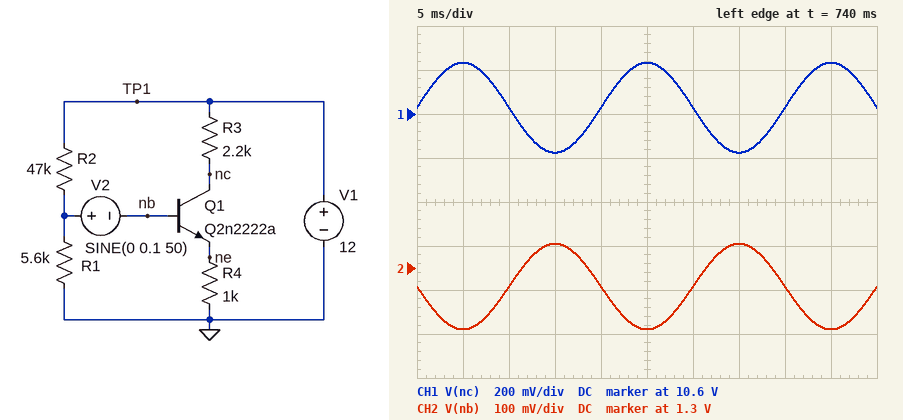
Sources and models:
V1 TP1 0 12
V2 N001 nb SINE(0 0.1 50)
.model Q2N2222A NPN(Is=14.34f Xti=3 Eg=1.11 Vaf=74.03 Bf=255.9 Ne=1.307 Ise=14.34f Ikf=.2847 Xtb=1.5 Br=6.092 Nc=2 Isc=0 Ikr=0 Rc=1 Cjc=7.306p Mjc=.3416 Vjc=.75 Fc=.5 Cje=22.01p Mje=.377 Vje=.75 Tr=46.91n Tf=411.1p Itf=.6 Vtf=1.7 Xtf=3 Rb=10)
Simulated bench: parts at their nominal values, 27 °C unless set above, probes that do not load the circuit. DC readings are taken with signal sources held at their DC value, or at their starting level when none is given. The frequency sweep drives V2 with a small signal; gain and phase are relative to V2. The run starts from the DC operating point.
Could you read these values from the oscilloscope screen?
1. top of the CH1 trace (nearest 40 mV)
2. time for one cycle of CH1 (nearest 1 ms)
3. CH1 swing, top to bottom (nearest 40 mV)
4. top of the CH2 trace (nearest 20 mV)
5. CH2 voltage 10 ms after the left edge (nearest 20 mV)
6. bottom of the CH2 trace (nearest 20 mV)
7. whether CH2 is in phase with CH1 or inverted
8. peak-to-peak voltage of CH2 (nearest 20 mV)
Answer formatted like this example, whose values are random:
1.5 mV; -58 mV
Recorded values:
10.84 V; 20 ms; 400 mV; 1.36 V; 1.26 V; 1.16 V; inverted; 200 mV
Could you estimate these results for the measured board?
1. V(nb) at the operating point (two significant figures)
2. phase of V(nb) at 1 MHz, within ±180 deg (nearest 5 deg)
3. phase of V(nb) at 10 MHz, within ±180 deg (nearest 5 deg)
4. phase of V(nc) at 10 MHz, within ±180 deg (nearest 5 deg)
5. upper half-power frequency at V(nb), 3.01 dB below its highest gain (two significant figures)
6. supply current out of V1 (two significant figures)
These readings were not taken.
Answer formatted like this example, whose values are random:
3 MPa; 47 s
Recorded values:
1.3 V; 160 deg; 130 deg; -90 deg; 2.6 MHz; 850 µA
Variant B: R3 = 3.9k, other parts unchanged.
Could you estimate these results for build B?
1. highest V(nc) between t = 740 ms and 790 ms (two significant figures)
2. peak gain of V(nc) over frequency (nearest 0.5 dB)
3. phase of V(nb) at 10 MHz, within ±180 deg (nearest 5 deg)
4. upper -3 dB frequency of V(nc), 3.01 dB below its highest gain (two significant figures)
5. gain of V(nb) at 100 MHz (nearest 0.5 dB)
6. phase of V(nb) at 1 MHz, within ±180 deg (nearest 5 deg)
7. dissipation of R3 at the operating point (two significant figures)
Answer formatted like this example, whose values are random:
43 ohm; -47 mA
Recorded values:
9.9 V; 11.0 dB; 140 deg; 1.7 MHz; -17.5 dB; 155 deg; 1.5 mW
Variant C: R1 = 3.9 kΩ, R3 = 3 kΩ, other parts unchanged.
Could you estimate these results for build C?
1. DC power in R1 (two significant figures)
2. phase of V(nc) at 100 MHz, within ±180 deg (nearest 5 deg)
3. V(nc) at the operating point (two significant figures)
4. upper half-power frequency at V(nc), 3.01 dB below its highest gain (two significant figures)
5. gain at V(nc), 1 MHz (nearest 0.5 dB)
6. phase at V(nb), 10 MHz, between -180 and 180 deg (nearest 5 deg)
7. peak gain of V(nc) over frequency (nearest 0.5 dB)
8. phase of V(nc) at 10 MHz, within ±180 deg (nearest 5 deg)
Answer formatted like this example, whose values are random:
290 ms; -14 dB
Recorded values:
210 µW; -170 deg; 11 V; 2.7 MHz; 8.0 dB; 135 deg; 8.5 dB; -95 deg
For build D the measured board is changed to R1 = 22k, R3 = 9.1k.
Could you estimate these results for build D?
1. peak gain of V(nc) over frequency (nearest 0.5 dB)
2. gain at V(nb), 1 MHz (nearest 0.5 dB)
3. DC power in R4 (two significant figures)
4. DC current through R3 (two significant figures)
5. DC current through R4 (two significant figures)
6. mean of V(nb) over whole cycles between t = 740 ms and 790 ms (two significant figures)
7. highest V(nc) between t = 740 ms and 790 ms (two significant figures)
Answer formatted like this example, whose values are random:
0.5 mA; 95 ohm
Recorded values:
-25.0 dB; -24.5 dB; 1.7 mW; 1.2 mA; 1.3 mA; 2.0 V; 1.3 V
